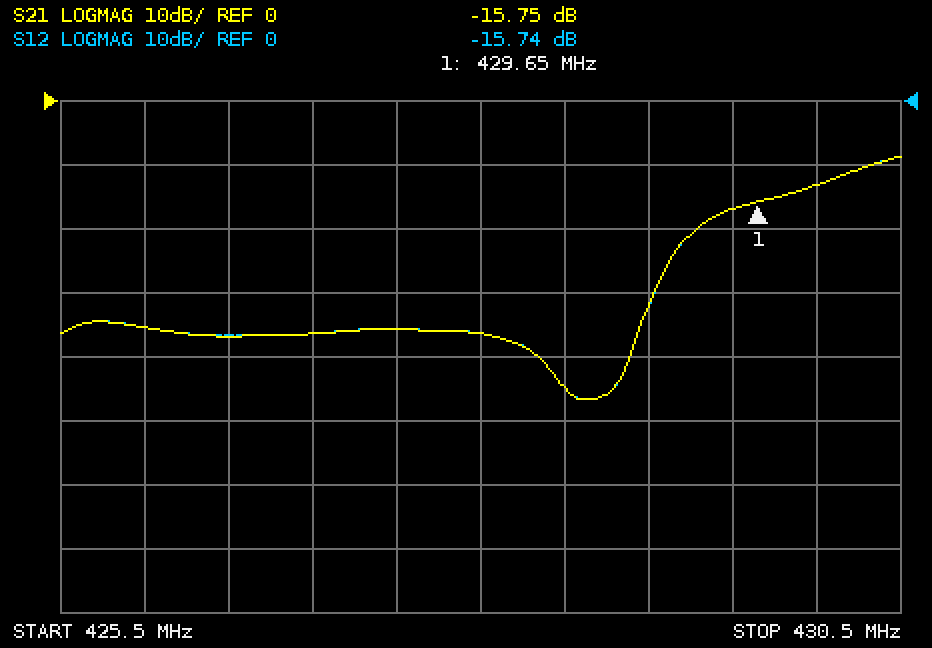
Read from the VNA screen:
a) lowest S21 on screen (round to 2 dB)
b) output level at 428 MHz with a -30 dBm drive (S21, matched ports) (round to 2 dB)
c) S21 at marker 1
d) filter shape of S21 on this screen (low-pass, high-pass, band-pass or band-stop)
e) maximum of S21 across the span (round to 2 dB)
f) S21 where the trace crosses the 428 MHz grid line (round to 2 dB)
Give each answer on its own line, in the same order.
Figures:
-46 dB
-66 dBm
-15.75 dB
high-pass
-8 dB
-36 dB
